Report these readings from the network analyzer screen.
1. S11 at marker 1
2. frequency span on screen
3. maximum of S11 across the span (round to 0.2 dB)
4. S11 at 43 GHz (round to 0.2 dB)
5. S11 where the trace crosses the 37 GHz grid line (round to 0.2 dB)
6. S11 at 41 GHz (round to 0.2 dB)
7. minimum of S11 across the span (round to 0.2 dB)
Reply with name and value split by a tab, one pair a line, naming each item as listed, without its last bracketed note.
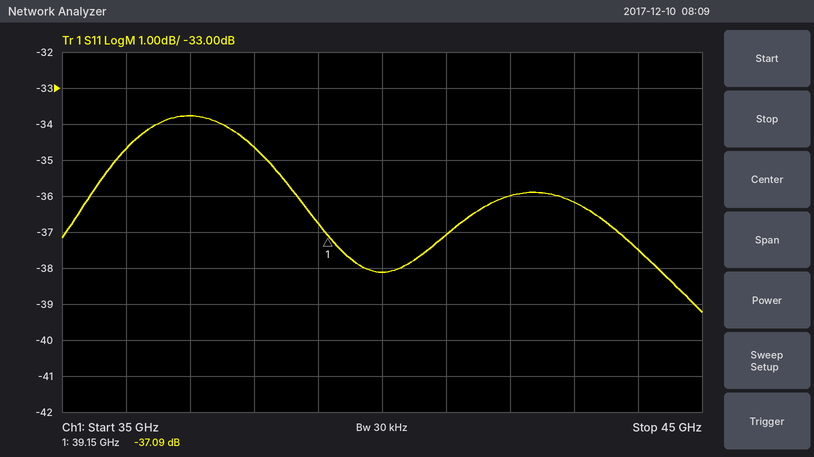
S11 at marker 1	-37.09 dB
frequency span on screen	10 GHz
maximum of S11 across the span	-33.8 dB
S11 at 43 GHz	-36.2 dB
S11 where the trace crosses the 37 GHz grid line	-33.8 dB
S11 at 41 GHz	-37.0 dB
minimum of S11 across the span	-39.2 dB
